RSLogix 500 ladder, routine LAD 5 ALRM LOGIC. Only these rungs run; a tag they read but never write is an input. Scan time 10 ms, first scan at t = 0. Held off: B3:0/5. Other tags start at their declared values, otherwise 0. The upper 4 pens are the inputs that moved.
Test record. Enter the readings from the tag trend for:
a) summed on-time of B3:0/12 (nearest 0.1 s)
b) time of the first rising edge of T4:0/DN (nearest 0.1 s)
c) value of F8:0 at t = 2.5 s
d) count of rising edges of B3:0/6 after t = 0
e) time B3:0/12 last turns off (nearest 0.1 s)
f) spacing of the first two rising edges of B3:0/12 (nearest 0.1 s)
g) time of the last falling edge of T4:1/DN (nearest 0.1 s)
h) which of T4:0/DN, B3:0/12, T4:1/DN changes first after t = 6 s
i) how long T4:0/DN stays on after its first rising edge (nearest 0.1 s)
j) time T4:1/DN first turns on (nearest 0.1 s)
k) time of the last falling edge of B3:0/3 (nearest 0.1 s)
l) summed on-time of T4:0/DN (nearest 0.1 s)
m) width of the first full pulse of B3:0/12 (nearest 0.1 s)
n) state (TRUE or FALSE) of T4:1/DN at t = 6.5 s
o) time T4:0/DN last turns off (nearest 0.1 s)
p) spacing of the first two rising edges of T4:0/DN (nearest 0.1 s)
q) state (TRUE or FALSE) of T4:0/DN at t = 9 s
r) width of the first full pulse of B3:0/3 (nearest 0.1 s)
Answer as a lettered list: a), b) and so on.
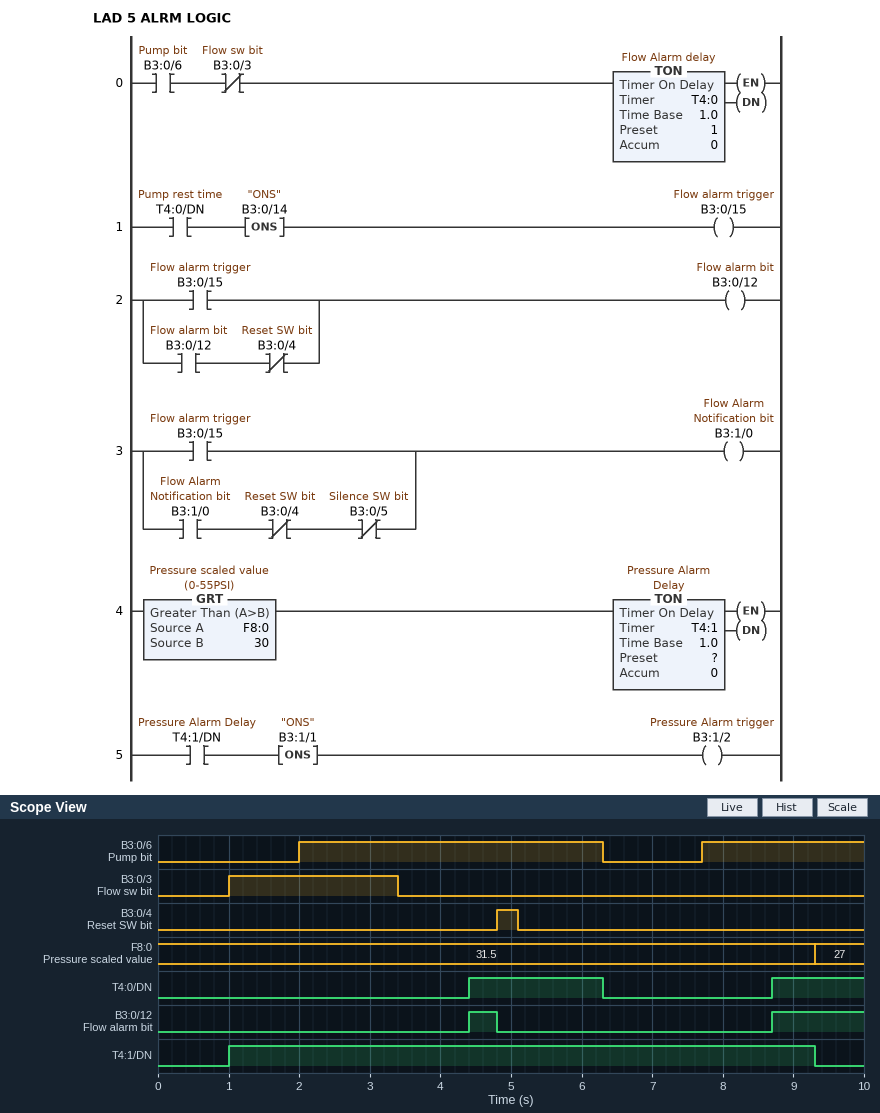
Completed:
a) 1.7 s
b) 4.4 s
c) 31.5
d) 2
e) 4.8 s
f) 4.3 s
g) 9.3 s
h) T4:0/DN
i) 1.9 s
j) 1.0 s
k) 3.4 s
l) 3.2 s
m) 0.4 s
n) TRUE
o) 6.3 s
p) 4.3 s
q) TRUE
r) 2.4 s
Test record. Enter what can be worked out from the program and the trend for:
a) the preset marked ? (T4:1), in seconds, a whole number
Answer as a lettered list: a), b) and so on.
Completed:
a) 1 s
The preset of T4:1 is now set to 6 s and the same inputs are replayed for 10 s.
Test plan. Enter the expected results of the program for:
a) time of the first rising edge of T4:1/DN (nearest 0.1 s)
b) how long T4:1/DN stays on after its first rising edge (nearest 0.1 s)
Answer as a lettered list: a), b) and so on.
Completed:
a) 6.0 s
b) 3.3 s
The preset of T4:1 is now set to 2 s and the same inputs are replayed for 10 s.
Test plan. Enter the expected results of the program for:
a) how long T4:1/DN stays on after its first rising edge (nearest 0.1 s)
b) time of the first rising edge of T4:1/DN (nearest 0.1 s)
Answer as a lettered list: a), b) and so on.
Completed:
a) 7.3 s
b) 2.0 s
